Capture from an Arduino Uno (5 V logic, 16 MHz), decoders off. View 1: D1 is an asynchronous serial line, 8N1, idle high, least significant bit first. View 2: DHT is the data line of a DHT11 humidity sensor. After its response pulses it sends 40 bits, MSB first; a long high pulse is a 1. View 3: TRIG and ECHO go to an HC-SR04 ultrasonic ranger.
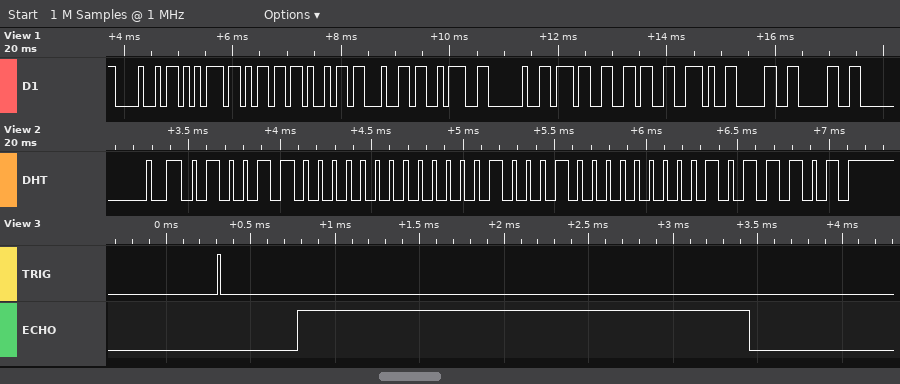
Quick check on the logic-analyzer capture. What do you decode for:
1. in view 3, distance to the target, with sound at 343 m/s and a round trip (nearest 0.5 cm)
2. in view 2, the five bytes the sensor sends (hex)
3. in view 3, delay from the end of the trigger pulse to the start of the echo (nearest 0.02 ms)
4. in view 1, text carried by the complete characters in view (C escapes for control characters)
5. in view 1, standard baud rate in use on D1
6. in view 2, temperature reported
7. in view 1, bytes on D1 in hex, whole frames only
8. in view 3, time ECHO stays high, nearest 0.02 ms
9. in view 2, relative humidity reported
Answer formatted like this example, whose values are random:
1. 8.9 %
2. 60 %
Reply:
1. 46 cm
2. 4C 00 11 00 5D
3. 0.46 ms
4. "Humid: 76.00"
5. 9600 baud
6. 17.0 °C
7. 0x48 0x75 0x6D 0x69 0x64 0x3A 0x20 0x37 0x36 0x2E 0x30 0x30
8. 2.68 ms
9. 76 %
